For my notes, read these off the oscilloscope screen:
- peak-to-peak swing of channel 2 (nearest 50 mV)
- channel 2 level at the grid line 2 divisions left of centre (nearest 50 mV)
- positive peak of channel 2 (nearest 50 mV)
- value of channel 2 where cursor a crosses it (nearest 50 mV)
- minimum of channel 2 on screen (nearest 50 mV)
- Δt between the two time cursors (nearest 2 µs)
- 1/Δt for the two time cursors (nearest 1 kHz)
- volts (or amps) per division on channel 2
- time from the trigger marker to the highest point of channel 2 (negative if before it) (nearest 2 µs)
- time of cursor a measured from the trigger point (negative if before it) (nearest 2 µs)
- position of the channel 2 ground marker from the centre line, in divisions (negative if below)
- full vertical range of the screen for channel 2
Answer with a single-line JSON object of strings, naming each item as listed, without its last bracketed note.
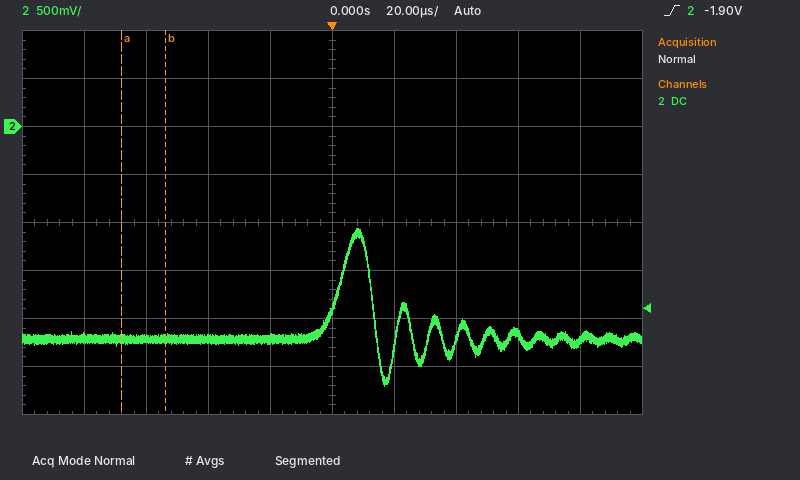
{"peak-to-peak swing of channel 2": "1.65 V", "channel 2 level at the grid line 2 divisions left of centre": "-2.20 V", "positive peak of channel 2": "-1.05 V", "value of channel 2 where cursor a crosses it": "-2.20 V", "minimum of channel 2 on screen": "-2.70 V", "Δt between the two time cursors": "14 µs", "1/Δt for the two time cursors": "71 kHz", "volts (or amps) per division on channel 2": "500 mV", "time from the trigger marker to the highest point of channel 2 (negative if before it)": "+8 µs", "time of cursor a measured from the trigger point (negative if before it)": "-68 µs", "position of the channel 2 ground marker from the centre line, in divisions": "+2.0 div", "full vertical range of the screen for channel 2": "4 V"}
